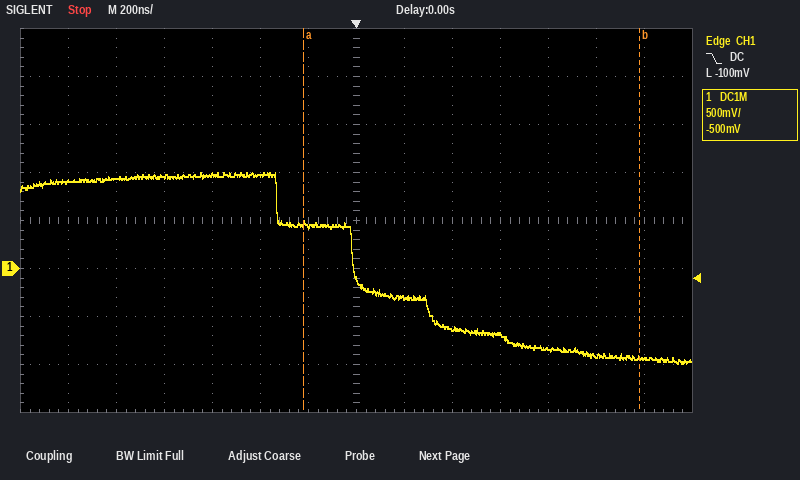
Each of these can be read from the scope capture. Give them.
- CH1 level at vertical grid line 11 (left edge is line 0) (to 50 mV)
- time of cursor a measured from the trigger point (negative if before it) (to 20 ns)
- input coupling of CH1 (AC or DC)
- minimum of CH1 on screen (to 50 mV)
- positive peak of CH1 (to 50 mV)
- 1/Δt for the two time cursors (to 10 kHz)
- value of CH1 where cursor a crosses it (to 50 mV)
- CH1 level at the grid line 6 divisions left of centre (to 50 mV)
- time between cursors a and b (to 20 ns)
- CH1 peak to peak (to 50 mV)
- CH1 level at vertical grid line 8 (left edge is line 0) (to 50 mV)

-850 mV
-220 ns
DC
-1.00 V
1.00 V
710 kHz
450 mV
900 mV
1.40 µs
2.00 V
-300 mV
